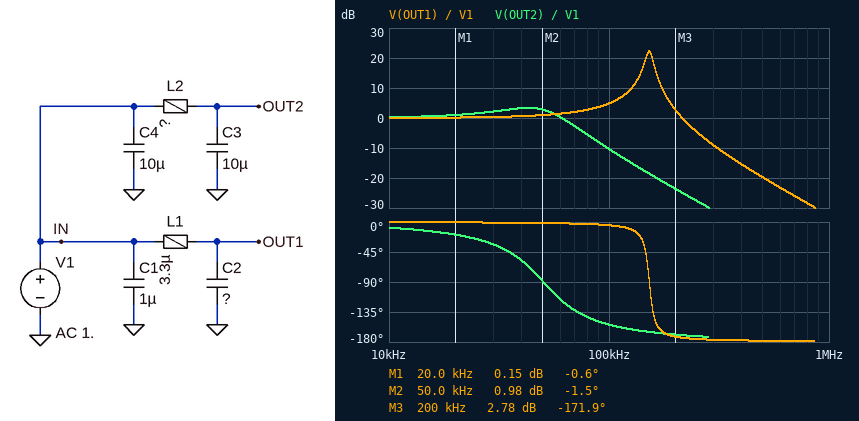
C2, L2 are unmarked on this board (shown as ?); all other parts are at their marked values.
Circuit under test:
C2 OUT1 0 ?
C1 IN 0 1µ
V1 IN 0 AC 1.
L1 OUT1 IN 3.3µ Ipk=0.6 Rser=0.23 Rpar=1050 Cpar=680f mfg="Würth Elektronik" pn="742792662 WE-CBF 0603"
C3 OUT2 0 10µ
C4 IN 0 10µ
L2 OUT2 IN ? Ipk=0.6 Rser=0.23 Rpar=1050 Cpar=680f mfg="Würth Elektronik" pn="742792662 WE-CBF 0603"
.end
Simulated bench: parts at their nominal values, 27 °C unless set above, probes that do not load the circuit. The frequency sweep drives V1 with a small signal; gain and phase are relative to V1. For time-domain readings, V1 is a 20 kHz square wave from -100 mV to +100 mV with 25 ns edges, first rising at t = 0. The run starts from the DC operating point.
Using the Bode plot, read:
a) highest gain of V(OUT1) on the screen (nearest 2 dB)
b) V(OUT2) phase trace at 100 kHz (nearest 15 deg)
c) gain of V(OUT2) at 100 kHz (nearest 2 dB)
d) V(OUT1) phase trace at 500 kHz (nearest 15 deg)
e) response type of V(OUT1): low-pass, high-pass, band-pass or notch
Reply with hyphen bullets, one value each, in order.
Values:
- 22 dB
- -150 deg
- -10 dB
- -180 deg
- low-pass
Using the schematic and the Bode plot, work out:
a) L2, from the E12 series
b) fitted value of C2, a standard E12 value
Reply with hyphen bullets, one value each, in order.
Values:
- 1 µH
- 330 nF
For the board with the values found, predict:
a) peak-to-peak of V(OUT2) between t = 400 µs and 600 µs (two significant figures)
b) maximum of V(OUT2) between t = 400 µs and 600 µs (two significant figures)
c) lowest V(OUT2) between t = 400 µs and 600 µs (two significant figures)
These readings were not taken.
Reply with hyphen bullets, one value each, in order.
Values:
- 310 mV
- 160 mV
- -160 mV
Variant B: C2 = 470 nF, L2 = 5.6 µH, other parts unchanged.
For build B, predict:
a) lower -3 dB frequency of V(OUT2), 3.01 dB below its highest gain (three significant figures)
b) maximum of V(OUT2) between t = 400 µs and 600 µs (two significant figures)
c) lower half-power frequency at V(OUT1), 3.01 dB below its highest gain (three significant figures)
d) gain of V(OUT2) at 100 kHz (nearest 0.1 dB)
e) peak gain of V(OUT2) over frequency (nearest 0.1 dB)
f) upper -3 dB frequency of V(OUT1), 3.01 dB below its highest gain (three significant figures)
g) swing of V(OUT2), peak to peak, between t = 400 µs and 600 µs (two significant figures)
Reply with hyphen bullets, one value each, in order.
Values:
- 17.1 kHz
- 400 mV
- 122 kHz
- -26.5 dB
- 10.3 dB
- 133 kHz
- 800 mV
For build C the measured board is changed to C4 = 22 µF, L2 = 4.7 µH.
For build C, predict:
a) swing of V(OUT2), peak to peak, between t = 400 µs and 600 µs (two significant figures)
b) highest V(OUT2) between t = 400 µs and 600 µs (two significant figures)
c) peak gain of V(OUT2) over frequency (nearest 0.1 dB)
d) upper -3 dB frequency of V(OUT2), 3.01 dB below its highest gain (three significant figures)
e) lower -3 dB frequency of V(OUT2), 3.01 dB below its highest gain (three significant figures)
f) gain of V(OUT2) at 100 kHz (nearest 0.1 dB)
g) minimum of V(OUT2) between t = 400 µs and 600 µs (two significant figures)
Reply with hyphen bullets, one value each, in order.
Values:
- 650 mV
- 320 mV
- 9.6 dB
- 26.2 kHz
- 18.2 kHz
- -24.9 dB
- -320 mV
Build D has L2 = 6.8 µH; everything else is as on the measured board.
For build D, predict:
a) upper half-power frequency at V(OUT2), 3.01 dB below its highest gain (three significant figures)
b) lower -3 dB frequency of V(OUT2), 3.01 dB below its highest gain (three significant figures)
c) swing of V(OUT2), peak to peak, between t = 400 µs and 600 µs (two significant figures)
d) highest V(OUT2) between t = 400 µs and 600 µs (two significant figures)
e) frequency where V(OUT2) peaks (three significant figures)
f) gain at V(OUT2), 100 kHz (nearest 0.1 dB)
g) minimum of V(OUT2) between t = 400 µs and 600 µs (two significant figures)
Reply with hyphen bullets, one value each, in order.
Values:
- 21.5 kHz
- 16.0 kHz
- 860 mV
- 430 mV
- 18.9 kHz
- -28.3 dB
- -430 mV
